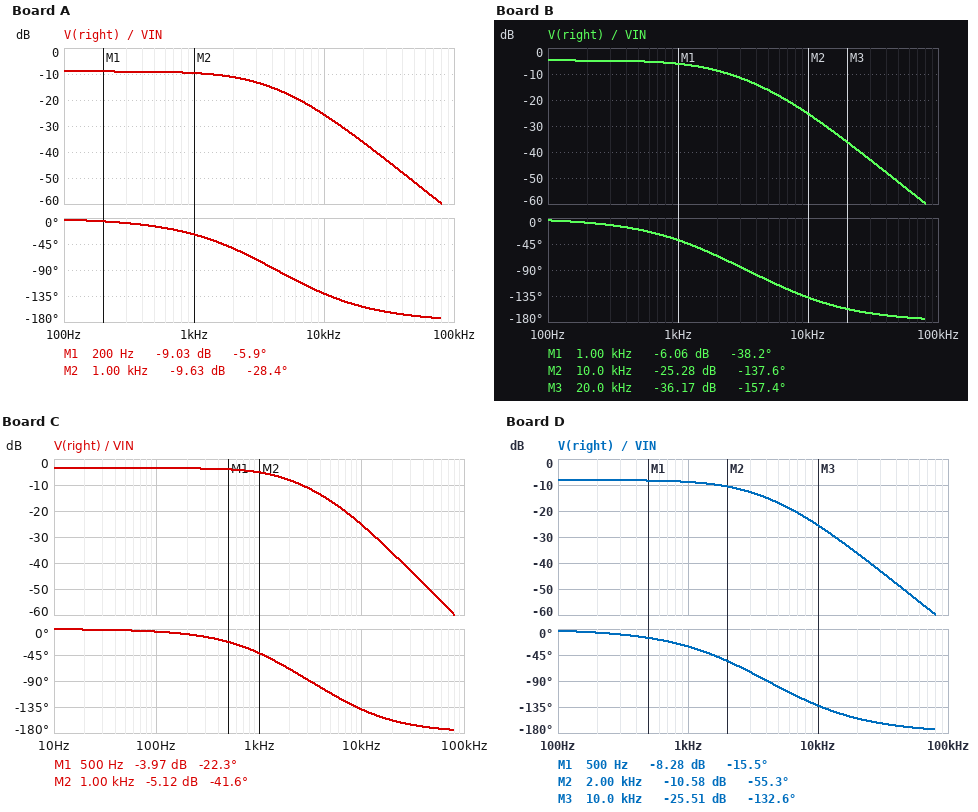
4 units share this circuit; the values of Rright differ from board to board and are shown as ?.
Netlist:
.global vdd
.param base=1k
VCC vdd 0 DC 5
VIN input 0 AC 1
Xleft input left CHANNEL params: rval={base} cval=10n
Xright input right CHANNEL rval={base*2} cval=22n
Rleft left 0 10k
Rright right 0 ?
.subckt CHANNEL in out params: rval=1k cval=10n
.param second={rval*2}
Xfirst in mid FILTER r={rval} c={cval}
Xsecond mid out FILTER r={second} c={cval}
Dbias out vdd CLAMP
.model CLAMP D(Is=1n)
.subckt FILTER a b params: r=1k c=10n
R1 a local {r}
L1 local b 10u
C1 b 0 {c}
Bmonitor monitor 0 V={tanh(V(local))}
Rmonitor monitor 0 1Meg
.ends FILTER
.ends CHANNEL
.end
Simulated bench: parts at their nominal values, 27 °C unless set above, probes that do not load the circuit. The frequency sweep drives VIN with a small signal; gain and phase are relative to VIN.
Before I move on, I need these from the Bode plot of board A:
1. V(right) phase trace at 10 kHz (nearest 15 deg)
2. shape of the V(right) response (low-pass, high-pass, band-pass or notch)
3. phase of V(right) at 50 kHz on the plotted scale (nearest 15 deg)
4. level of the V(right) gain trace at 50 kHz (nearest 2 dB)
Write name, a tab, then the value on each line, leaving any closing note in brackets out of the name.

V(right) phase trace at 10 kHz	-135 deg
shape of the V(right) response	low-pass
phase of V(right) at 50 kHz on the plotted scale	-165 deg
level of the V(right) gain trace at 50 kHz	-52 dB
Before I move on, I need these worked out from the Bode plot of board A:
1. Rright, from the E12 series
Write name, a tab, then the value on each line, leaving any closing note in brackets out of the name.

Rright, from the E12 series	3.3 kΩ
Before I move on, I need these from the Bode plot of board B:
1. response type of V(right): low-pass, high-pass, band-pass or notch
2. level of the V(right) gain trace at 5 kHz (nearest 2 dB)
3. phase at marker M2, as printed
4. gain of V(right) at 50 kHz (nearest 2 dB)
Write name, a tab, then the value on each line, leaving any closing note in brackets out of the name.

response type of V(right): low-pass, high-pass, band-pass or notch	low-pass
level of the V(right) gain trace at 5 kHz	-16 dB
phase at marker M2, as printed	-137.6 deg
gain of V(right) at 50 kHz	-52 dB
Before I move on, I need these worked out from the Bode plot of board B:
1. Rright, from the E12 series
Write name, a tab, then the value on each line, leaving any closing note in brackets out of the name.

Rright, from the E12 series	8.2 kΩ
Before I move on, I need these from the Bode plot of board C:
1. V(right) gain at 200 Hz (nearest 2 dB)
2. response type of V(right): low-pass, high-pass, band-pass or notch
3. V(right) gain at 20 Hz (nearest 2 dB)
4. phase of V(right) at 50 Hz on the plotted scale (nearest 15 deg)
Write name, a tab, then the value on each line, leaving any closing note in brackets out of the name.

V(right) gain at 200 Hz	-4 dB
response type of V(right): low-pass, high-pass, band-pass or notch	low-pass
V(right) gain at 20 Hz	-4 dB
phase of V(right) at 50 Hz on the plotted scale	0 deg
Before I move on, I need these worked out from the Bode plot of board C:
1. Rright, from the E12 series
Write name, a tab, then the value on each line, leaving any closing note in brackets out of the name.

Rright, from the E12 series	12 kΩ
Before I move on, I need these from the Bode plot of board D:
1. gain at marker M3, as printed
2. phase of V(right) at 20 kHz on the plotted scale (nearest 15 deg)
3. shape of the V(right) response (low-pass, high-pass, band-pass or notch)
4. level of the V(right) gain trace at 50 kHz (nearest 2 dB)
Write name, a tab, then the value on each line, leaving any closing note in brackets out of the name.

gain at marker M3, as printed	-25.51 dB
phase of V(right) at 20 kHz on the plotted scale	-150 deg
shape of the V(right) response	low-pass
level of the V(right) gain trace at 50 kHz	-52 dB
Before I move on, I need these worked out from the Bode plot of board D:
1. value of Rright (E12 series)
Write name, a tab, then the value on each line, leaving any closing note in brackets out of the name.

value of Rright	3.9 kΩ
